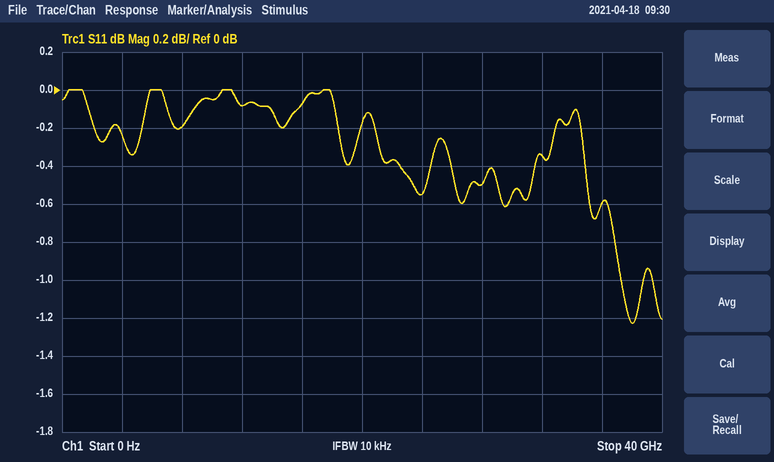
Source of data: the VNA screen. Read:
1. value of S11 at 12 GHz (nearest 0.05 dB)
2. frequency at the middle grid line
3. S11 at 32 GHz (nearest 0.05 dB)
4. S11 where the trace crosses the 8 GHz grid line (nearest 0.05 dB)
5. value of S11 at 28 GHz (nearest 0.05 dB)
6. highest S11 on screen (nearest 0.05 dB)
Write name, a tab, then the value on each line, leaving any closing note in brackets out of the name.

value of S11 at 12 GHz	-0.10 dB
frequency at the middle grid line	20 GHz
S11 at 32 GHz	-0.35 dB
S11 where the trace crosses the 8 GHz grid line	-0.20 dB
value of S11 at 28 GHz	-0.50 dB
highest S11 on screen	0.00 dB
